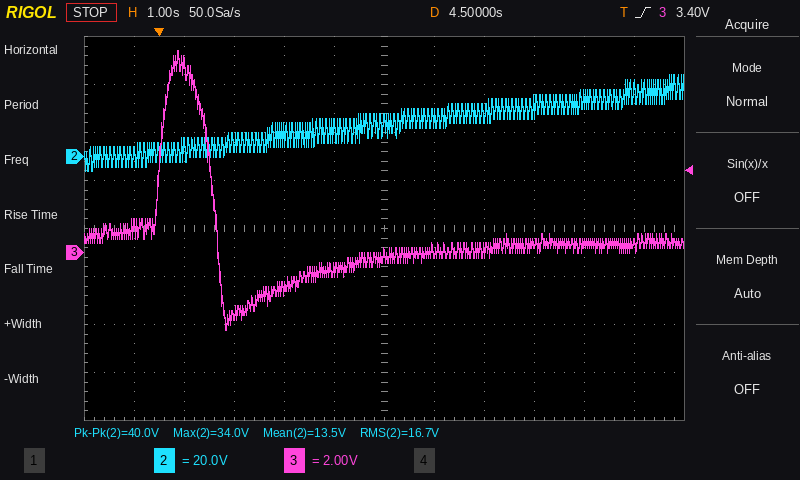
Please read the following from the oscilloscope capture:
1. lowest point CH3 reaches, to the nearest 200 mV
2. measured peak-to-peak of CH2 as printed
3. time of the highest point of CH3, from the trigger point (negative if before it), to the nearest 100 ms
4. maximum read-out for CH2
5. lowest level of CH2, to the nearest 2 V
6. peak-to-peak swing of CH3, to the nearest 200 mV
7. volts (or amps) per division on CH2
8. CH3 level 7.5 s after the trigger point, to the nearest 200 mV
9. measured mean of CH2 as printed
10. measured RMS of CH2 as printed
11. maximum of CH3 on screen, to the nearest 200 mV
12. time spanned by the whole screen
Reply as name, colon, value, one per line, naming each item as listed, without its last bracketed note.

lowest point CH3 reaches, to the nearest 200 mV: -3.2 V
measured peak-to-peak of CH2 as printed: 40.0 V
time of the highest point of CH3, from the trigger point (negative if before it), to the nearest 100 ms: +400 ms
maximum read-out for CH2: 34.0 V
lowest level of CH2, to the nearest 2 V: -6 V
peak-to-peak swing of CH3, to the nearest 200 mV: 11.6 V
volts (or amps) per division on CH2: 20 V
CH3 level 7.5 s after the trigger point, to the nearest 200 mV: 400 mV
measured mean of CH2 as printed: 13.5 V
measured RMS of CH2 as printed: 16.7 V
maximum of CH3 on screen, to the nearest 200 mV: 8.4 V
time spanned by the whole screen: 12 s
